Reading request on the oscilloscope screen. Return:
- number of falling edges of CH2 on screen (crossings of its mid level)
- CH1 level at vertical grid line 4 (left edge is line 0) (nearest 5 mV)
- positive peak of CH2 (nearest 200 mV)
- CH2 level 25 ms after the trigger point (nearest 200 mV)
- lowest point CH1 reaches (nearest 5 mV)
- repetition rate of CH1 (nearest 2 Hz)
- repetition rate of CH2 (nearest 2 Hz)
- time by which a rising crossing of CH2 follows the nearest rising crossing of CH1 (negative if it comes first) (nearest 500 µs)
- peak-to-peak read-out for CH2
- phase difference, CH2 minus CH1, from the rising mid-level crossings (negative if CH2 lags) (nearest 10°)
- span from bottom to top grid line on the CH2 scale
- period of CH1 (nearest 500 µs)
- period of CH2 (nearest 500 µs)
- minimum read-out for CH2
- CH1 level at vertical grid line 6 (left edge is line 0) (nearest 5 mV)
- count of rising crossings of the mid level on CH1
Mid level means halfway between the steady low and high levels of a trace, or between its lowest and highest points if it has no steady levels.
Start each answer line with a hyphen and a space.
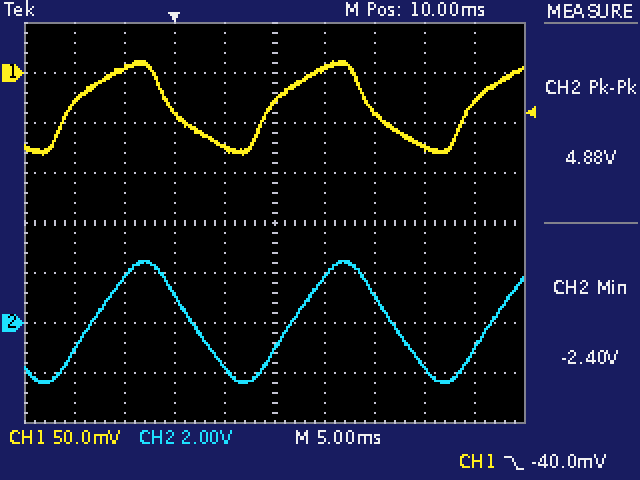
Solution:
- 2
- -75 mV
- 2.4 V
- -1.8 V
- -80 mV
- 50 Hz
- 50 Hz
- +2.0 ms
- 4.88 V
- -40°
- 16 V
- 20.0 ms
- 20.0 ms
- -2.40 V
- 5 mV
- 3
